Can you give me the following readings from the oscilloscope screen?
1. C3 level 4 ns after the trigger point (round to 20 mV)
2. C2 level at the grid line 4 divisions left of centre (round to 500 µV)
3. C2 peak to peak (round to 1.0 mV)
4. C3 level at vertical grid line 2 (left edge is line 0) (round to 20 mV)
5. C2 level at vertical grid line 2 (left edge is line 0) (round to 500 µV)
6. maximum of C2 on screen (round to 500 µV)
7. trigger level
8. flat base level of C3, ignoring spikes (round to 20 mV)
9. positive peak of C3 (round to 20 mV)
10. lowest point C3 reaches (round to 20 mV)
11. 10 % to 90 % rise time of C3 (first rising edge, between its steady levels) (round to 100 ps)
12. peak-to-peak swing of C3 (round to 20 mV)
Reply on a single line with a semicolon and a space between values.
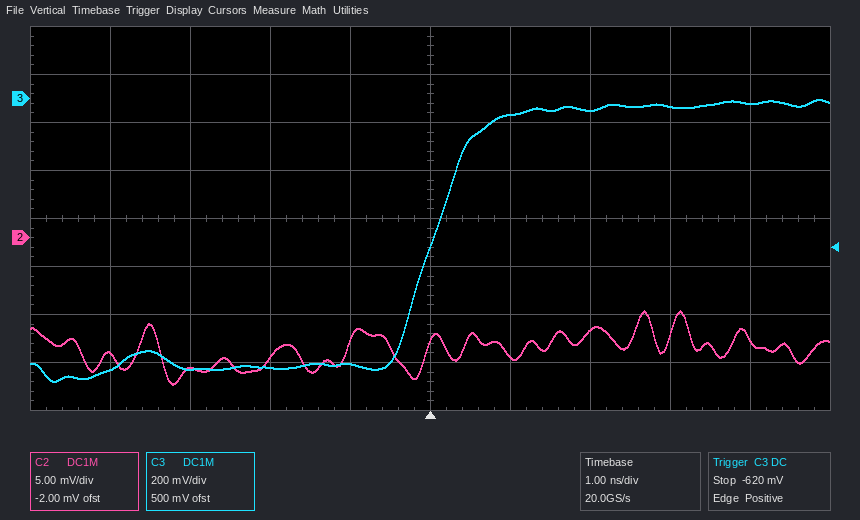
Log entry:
-20 mV; -12.0 mV; 8.0 mV; -1.12 V; -13.5 mV; -7.5 mV; -620 mV; -1.12 V; 0 mV; -1.18 V; 1.0 ns; 1.18 V
